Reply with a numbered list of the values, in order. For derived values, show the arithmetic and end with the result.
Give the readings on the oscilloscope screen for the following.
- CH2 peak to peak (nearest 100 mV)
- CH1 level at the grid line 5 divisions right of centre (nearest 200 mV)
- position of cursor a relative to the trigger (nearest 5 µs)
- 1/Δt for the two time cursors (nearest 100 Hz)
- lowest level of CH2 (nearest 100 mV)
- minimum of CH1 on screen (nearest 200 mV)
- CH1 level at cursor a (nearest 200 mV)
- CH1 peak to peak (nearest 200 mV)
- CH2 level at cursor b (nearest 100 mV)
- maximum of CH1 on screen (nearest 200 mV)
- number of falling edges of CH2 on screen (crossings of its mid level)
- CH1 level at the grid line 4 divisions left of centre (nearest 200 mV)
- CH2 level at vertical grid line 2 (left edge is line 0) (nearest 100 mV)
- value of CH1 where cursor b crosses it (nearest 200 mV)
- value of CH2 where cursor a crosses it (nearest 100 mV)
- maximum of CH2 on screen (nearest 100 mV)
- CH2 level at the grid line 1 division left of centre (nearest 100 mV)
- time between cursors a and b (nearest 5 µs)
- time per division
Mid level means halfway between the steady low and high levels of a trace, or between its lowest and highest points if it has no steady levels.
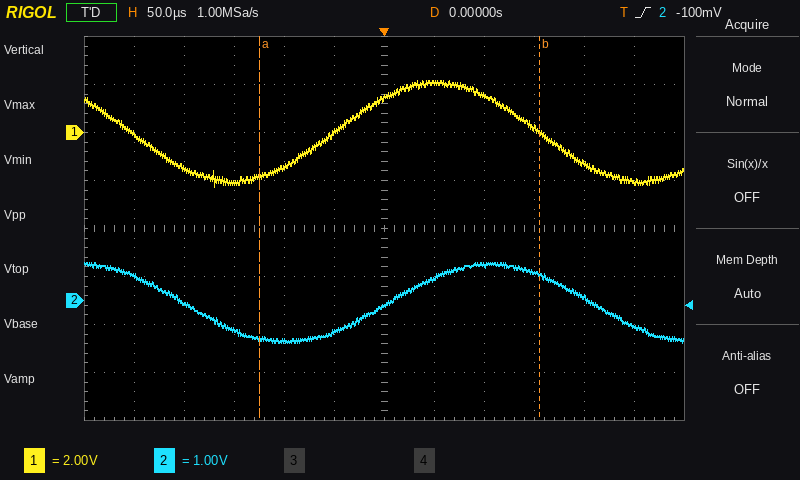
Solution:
1. 800 mV − (-900 mV) = 1.7 V
2. -2.0 V
3. -125 µs
4. 1 / 280 µs ≈ 3.6 kHz
5. -900 mV
6. -2.2 V
7. -1.8 V
8. 2.2 V − (-2.2 V) = 4.4 V
9. 500 mV
10. 2.2 V
11. 2
12. -1.4 V
13. -100 mV
14. 0.0 V
15. -800 mV
16. 800 mV
17. -700 mV
18. 280 µs
19. 50 µs
